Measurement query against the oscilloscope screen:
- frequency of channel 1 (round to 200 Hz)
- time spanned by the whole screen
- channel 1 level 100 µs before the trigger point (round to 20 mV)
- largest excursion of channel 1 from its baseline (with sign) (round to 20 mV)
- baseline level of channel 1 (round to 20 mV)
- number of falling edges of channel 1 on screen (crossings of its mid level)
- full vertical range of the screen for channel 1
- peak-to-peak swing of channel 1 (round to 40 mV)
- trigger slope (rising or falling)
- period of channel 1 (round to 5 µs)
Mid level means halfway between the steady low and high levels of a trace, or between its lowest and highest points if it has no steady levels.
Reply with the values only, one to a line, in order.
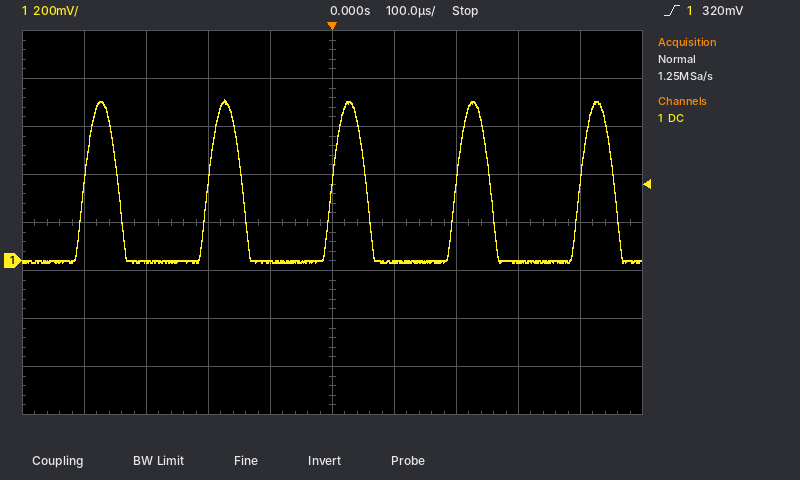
5.0 kHz
1 ms
0 mV
+680 mV
0 mV
5
1.6 V
680 mV
rising
200 µs
